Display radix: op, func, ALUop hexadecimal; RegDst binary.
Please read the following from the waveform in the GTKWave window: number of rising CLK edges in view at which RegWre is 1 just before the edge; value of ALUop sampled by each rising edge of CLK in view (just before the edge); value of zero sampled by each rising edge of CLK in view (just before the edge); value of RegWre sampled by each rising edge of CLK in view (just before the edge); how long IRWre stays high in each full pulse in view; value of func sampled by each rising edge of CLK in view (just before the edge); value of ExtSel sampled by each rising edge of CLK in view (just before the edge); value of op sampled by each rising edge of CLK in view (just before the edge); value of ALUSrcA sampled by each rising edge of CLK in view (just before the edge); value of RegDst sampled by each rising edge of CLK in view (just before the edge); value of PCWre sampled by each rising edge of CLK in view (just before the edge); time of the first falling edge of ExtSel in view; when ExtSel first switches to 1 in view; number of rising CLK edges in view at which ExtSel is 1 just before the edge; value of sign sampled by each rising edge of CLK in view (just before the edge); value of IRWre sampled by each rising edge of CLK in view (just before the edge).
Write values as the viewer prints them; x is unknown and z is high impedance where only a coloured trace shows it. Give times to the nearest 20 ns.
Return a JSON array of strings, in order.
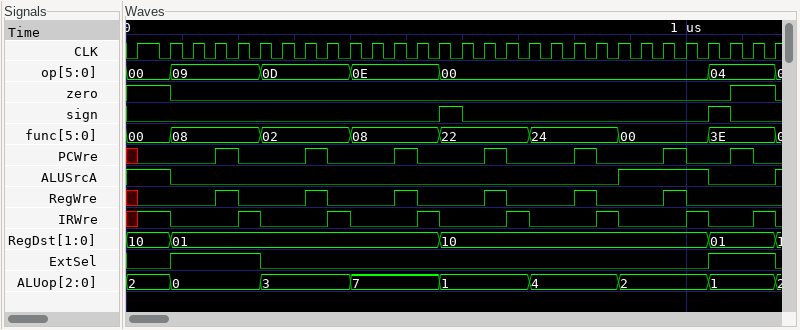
["6", "2, 2, 0, 0, 0, 0, 3, 3, 3, 3, 7, 7, 7, 7, 1, 1, 1, 1, 4, 4, 4, 4, 2, 2, 2, 2, 1, 1, 1", "1 1 0 0 0 0 0 0 0 0 0 0 0 0 0 0 0 0 0 0 0 0 0 0 0 0 0 1 1", "x 0 0 0 1 0 0 0 1 0 0 0 1 0 0 0 1 0 0 0 1 0 0 0 1 0 0 0 0", "40 ns, 40 ns, 40 ns, 40 ns, 40 ns, 40 ns, 40 ns", "00, 00, 08, 08, 08, 08, 02, 02, 02, 02, 08, 08, 08, 08, 22, 22, 22, 22, 24, 24, 24, 24, 00, 00, 00, 00, 3E, 3E, 3E", "0 0 1 1 1 1 0 0 0 0 0 0 0 0 0 0 0 0 0 0 0 0 0 0 0 0 1 1 1", "00, 00, 09, 09, 09, 09, 0D, 0D, 0D, 0D, 0E, 0E, 0E, 0E, 00, 00, 00, 00, 00, 00, 00, 00, 00, 00, 00, 00, 04, 04, 04", "1 1 0 0 0 0 0 0 0 0 0 0 0 0 0 0 0 0 0 0 0 0 1 1 1 1 0 0 0", "10, 10, 01, 01, 01, 01, 01, 01, 01, 01, 01, 01, 01, 01, 10, 10, 10, 10, 10, 10, 10, 10, 10, 10, 10, 10, 01, 01, 01", "x 0 0 0 1 0 0 0 1 0 0 0 1 0 0 0 1 0 0 0 1 0 0 0 1 0 0 1 0", "240 ns", "80 ns", "7", "0 0 0 0 0 0 0 0 0 0 0 0 0 0 1 0 0 0 0 0 0 0 0 0 0 0 1 0 0", "x 1 0 0 0 1 0 0 0 1 0 0 0 1 0 0 0 1 0 0 0 1 0 0 0 1 0 0 1"]
